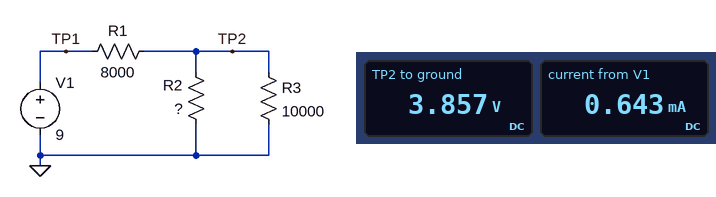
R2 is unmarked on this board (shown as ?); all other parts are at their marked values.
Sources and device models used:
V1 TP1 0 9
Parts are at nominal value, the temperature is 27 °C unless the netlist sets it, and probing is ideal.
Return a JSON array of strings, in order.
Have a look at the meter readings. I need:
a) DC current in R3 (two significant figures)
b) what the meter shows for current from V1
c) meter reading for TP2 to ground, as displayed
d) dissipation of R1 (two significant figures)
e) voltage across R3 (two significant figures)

["390 µA", "0.643 mA", "3.857 V", "3.3 mW", "3.9 V"]
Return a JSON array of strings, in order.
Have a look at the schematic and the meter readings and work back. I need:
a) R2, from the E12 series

["15 kΩ"]
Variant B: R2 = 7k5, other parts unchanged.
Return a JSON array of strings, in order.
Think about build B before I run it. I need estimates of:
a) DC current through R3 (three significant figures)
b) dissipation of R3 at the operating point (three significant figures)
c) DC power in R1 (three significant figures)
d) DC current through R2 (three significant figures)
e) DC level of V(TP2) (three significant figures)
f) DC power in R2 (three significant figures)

["314 µA", "986 µW", "4.29 mW", "419 µA", "3.14 V", "1.31 mW"]
